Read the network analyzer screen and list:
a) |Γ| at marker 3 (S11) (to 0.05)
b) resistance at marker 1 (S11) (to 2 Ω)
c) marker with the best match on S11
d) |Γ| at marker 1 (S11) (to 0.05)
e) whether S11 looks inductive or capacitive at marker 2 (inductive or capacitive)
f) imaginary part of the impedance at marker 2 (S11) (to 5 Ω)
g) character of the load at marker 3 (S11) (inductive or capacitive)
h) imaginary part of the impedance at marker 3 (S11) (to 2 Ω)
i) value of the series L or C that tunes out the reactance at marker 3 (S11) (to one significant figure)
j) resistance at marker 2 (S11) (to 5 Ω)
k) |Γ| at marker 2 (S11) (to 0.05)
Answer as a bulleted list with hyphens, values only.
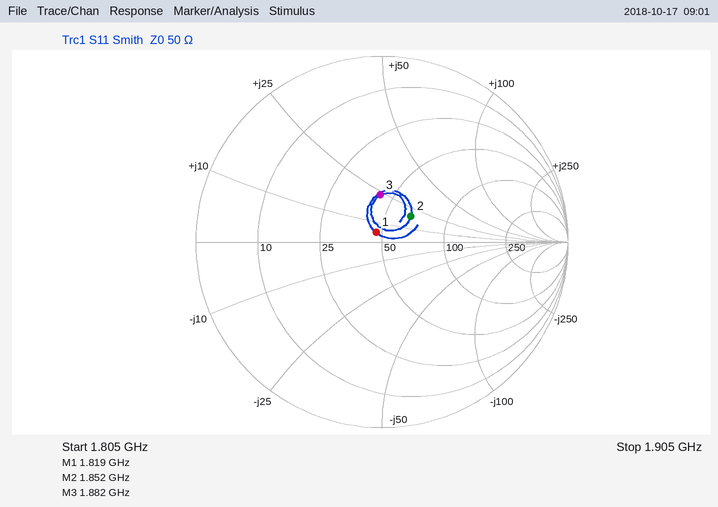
- 0.25
- 46 Ω
- marker 1
- 0.05
- inductive
- +20 Ω
- inductive
- +24 Ω
- 4 pF
- 65 Ω
- 0.20
